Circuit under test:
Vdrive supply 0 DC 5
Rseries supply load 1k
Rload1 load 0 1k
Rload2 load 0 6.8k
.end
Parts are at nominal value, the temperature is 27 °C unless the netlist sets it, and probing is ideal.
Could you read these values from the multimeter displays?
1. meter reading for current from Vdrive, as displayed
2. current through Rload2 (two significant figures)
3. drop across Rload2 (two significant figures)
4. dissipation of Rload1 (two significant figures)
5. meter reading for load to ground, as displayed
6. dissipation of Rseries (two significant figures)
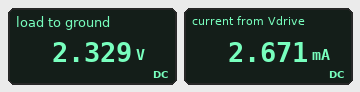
2.671 mA
340 µA
2.3 V
5.4 mW
2.329 V
7.1 mW
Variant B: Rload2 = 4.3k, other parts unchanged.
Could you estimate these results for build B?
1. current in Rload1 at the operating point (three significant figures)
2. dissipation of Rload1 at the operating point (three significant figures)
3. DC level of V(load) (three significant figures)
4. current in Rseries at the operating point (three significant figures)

2.24 mA
5.02 mW
2.24 V
2.76 mA
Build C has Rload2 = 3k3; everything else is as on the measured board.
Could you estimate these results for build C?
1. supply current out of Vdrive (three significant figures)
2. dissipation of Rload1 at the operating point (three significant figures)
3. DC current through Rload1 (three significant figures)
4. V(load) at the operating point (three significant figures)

2.83 mA
4.71 mW
2.17 mA
2.17 V
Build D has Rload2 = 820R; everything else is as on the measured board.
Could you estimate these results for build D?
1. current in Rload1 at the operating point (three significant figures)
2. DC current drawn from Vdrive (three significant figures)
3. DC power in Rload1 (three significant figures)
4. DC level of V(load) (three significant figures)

1.55 mA
3.45 mA
2.41 mW
1.55 V
